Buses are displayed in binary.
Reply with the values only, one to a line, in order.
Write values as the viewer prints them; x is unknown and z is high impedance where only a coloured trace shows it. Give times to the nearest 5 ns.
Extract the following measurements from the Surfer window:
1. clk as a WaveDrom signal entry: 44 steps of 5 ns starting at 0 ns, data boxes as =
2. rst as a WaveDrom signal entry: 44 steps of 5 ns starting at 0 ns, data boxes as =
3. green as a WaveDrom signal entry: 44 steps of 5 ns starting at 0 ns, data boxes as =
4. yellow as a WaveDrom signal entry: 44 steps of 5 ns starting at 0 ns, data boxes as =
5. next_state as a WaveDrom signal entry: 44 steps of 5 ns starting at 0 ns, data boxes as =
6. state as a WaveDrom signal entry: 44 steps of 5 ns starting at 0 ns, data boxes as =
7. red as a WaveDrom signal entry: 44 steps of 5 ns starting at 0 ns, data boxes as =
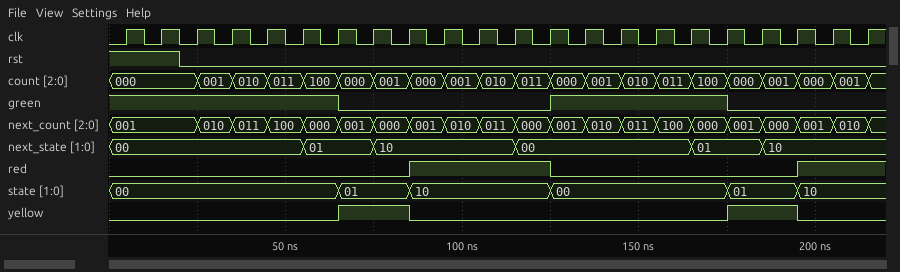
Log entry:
{name: 'clk', wave: '01010101010101010101010101010101010101010101'}
{name: 'rst', wave: '1...0.......................................'}
{name: 'green', wave: '1............0...........1.........0........'}
{name: 'yellow', wave: '0............1...0.................1...0....'}
{name: 'next_state', wave: '=..........=...=.......=.........=...=......', data: '00 01 10 00 01 10'}
{name: 'state', wave: '=............=...=.......=.........=...=....', data: '00 01 10 00 01 10'}
{name: 'red', wave: '0................1.......0.............1....'}
